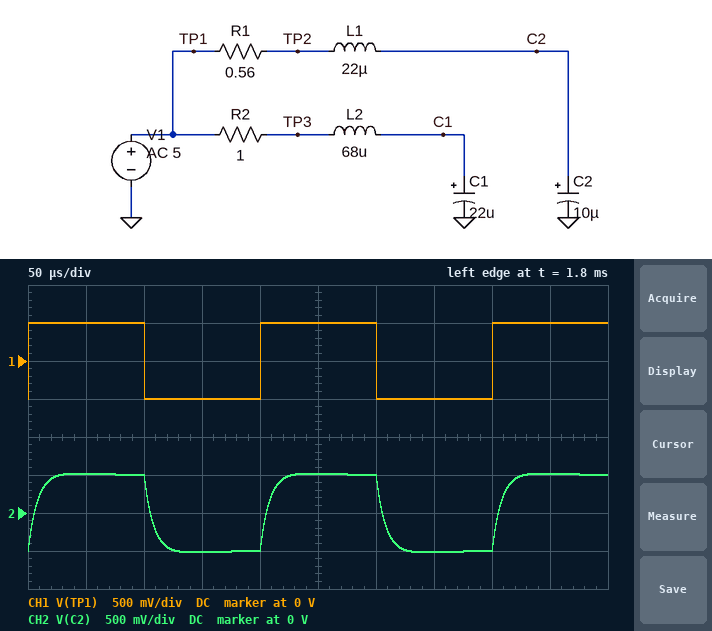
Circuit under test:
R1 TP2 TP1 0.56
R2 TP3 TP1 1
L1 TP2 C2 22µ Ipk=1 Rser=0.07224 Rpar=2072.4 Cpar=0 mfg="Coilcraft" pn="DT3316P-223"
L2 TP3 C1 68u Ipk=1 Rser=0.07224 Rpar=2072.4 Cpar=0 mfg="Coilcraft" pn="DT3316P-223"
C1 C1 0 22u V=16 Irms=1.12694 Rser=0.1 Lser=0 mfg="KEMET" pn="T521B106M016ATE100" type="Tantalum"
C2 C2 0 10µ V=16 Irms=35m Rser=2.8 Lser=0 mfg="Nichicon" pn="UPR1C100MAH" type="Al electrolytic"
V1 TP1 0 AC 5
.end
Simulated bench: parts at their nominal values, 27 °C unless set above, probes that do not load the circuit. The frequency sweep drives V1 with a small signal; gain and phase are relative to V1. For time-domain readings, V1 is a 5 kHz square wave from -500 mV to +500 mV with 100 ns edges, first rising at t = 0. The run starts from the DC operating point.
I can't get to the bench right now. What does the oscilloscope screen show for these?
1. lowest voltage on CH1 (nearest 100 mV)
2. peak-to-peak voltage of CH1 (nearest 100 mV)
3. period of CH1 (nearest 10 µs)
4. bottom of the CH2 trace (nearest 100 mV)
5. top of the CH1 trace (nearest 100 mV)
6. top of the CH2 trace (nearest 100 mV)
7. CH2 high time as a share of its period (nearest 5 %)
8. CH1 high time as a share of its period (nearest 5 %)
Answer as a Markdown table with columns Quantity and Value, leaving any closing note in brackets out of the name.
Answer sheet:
| Quantity | Value |
|---|---|
| lowest voltage on CH1 | -500 mV |
| peak-to-peak voltage of CH1 | 1.0 V |
| period of CH1 | 200 µs |
| bottom of the CH2 trace | -500 mV |
| top of the CH1 trace | 500 mV |
| top of the CH2 trace | 500 mV |
| CH2 high time as a share of its period | 50 % |
| CH1 high time as a share of its period | 50 % |
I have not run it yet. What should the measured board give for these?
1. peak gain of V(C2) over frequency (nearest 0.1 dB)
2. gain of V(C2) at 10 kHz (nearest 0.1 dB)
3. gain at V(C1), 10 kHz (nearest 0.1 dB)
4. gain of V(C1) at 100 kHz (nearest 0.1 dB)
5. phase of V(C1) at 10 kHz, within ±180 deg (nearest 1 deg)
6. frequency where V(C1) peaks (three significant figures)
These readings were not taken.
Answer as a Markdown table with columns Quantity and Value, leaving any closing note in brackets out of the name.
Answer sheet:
| Quantity | Value |
|---|---|
| peak gain of V(C2) over frequency | 0 dB |
| gain of V(C2) at 10 kHz | -0.6 dB |
| gain at V(C1), 10 kHz | -14.2 dB |
| gain of V(C1) at 100 kHz | -50.8 dB |
| phase of V(C1) at 10 kHz, within ±180 deg | -154 deg |
| frequency where V(C1) peaks | 3.63 kHz |
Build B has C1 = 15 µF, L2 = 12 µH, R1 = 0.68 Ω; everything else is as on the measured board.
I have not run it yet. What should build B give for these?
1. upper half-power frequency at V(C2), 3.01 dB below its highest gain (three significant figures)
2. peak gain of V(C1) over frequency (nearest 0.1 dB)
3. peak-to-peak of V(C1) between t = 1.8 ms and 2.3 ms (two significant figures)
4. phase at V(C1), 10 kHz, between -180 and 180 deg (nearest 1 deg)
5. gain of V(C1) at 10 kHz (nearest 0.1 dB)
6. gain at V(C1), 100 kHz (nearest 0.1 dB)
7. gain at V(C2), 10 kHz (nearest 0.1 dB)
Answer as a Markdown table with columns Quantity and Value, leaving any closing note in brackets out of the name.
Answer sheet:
| Quantity | Value |
|---|---|
| upper half-power frequency at V(C2), 3.01 dB below its highest gain | 20.5 kHz |
| peak gain of V(C1) over frequency | 0.1 dB |
| peak-to-peak of V(C1) between t = 1.8 ms and 2.3 ms | 1.1 V |
| phase at V(C1), 10 kHz, between -180 and 180 deg | -70 deg |
| gain of V(C1) at 10 kHz | -1.1 dB |
| gain at V(C1), 100 kHz | -34.3 dB |
| gain at V(C2), 10 kHz | -0.9 dB |
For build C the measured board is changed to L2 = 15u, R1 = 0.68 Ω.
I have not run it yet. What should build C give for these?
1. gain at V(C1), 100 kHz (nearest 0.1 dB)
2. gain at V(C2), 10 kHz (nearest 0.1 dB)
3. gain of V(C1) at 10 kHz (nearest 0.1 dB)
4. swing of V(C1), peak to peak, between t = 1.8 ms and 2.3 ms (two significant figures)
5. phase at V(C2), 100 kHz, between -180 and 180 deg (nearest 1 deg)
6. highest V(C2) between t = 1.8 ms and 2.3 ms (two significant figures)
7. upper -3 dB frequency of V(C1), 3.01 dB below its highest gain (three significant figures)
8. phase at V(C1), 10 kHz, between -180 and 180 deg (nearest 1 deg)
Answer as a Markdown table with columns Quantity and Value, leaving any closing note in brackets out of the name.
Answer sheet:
| Quantity | Value |
|---|---|
| gain at V(C1), 100 kHz | -37.7 dB |
| gain at V(C2), 10 kHz | -0.9 dB |
| gain of V(C1) at 10 kHz | -4.3 dB |
| swing of V(C1), peak to peak, between t = 1.8 ms and 2.3 ms | 1.1 V |
| phase at V(C2), 100 kHz, between -180 and 180 deg | -78 deg |
| highest V(C2) between t = 1.8 ms and 2.3 ms | 500 mV |
| upper -3 dB frequency of V(C1), 3.01 dB below its highest gain | 8.79 kHz |
| phase at V(C1), 10 kHz, between -180 and 180 deg | -93 deg |
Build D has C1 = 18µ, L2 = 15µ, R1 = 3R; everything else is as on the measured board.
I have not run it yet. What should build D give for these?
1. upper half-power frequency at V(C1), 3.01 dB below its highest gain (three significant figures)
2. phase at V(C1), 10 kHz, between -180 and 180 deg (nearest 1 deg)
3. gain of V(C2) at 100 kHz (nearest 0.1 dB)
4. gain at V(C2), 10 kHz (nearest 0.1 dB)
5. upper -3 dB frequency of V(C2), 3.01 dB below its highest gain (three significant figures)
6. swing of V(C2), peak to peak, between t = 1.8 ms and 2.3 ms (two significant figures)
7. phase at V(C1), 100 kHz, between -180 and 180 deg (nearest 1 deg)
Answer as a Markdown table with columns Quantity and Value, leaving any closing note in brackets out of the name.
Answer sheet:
| Quantity | Value |
|---|---|
| upper half-power frequency at V(C1), 3.01 dB below its highest gain | 10.5 kHz |
| phase at V(C1), 10 kHz, between -180 and 180 deg | -86 deg |
| gain of V(C2) at 100 kHz | -14.5 dB |
| gain at V(C2), 10 kHz | -5.2 dB |
| upper -3 dB frequency of V(C2), 3.01 dB below its highest gain | 4.15 kHz |
| swing of V(C2), peak to peak, between t = 1.8 ms and 2.3 ms | 850 mV |
| phase at V(C1), 100 kHz, between -180 and 180 deg | -124 deg |
